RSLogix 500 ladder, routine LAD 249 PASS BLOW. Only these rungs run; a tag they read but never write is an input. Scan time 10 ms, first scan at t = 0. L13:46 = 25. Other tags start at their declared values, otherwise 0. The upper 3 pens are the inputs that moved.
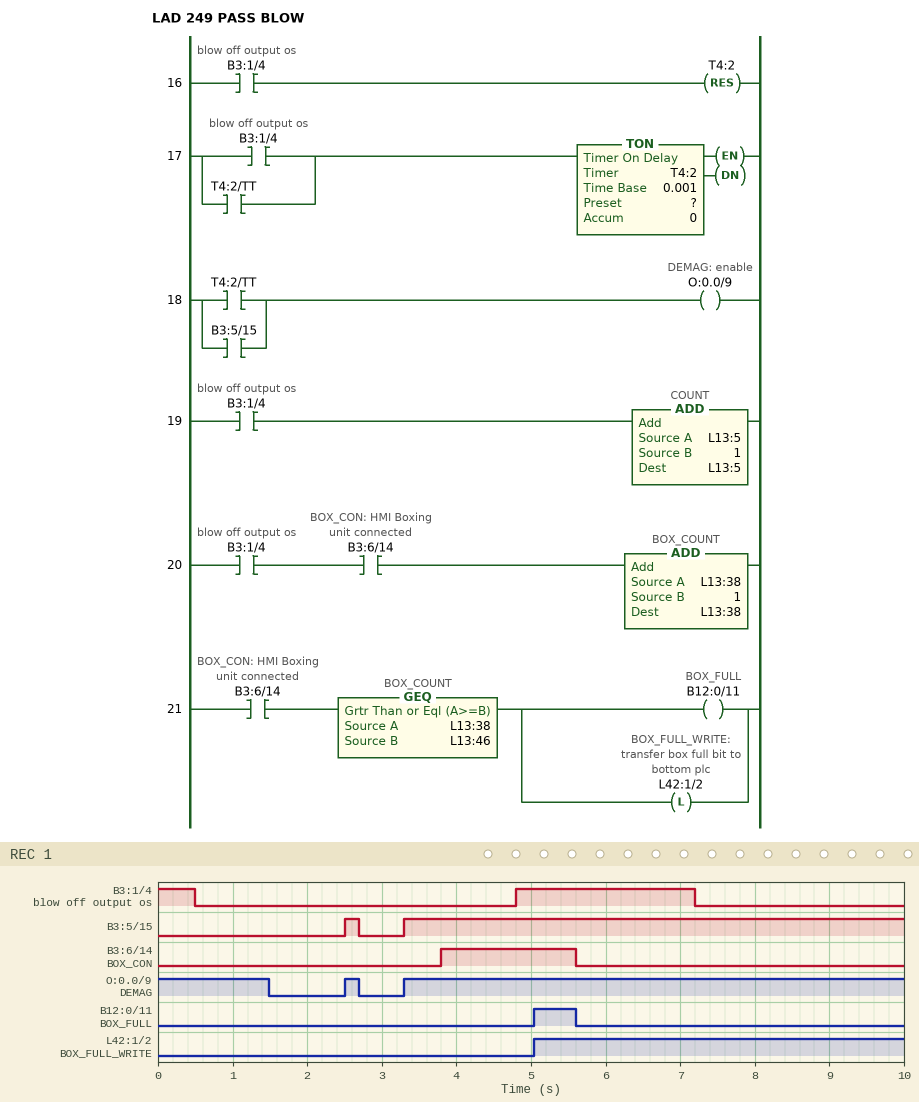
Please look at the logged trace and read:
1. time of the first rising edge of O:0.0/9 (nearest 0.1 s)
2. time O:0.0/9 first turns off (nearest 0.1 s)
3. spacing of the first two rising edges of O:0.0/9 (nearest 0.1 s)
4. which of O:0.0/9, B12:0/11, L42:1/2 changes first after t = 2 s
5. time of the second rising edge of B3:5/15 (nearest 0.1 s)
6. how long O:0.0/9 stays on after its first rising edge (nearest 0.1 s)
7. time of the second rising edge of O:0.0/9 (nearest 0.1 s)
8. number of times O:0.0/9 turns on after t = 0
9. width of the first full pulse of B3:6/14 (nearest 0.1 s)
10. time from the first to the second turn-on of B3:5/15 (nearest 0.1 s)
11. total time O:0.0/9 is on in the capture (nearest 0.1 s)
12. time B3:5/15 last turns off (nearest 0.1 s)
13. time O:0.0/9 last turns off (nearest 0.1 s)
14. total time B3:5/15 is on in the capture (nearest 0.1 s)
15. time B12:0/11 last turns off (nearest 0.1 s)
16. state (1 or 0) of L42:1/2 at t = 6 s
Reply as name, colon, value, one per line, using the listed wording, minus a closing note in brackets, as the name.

time of the first rising edge of O:0.0/9: 2.5 s
time O:0.0/9 first turns off: 1.5 s
spacing of the first two rising edges of O:0.0/9: 0.8 s
which of O:0.0/9, B12:0/11, L42:1/2 changes first after t = 2 s: O:0.0/9
time of the second rising edge of B3:5/15: 3.3 s
how long O:0.0/9 stays on after its first rising edge: 0.2 s
time of the second rising edge of O:0.0/9: 3.3 s
number of times O:0.0/9 turns on after t = 0: 2
width of the first full pulse of B3:6/14: 1.8 s
time from the first to the second turn-on of B3:5/15: 0.8 s
total time O:0.0/9 is on in the capture: 8.4 s
time B3:5/15 last turns off: 2.7 s
time O:0.0/9 last turns off: 2.7 s
total time B3:5/15 is on in the capture: 6.9 s
time B12:0/11 last turns off: 5.6 s
state (1 or 0) of L42:1/2 at t = 6 s: 1
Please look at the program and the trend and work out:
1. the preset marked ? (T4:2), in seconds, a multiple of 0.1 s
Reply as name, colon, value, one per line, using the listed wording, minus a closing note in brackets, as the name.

the preset marked ? (T4:2), in seconds, a multiple of 0.1 s: 1.0 s
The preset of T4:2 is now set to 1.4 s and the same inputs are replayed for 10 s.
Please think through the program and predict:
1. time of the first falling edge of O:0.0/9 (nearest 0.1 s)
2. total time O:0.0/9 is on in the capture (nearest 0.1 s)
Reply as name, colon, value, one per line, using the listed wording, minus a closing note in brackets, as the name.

time of the first falling edge of O:0.0/9: 1.9 s
total time O:0.0/9 is on in the capture: 8.8 s
